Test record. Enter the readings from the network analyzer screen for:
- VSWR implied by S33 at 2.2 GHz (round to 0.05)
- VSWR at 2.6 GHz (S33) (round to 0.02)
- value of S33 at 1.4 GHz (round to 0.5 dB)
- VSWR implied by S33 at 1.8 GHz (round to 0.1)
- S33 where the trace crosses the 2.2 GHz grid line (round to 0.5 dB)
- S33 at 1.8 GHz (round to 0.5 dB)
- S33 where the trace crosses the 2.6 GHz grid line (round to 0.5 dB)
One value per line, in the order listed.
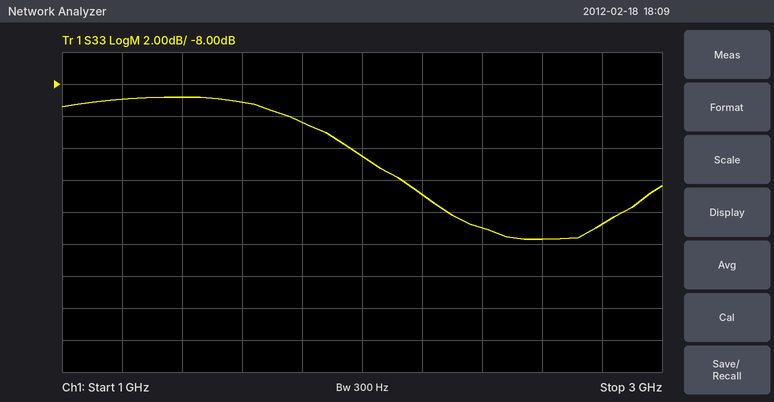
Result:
1.45
1.30
-9.0 dB
1.9
-15.0 dB
-10.5 dB
-17.5 dB
